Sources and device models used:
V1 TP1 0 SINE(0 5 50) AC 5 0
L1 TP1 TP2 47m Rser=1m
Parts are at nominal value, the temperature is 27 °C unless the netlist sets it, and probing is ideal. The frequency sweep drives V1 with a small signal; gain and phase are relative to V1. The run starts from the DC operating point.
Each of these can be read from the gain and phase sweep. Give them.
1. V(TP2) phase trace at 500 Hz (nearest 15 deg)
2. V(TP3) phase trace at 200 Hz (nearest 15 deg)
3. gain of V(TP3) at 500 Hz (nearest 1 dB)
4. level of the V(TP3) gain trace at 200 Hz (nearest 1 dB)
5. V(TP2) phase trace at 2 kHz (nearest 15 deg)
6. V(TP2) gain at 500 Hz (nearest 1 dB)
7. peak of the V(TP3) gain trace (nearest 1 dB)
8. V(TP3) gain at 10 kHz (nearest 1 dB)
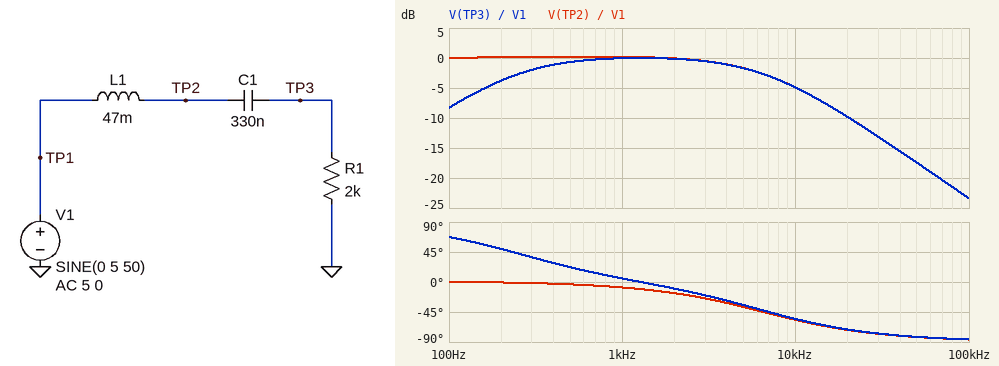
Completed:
0 deg
45 deg
-1 dB
-4 dB
-15 deg
0 dB
0 dB
-5 dB
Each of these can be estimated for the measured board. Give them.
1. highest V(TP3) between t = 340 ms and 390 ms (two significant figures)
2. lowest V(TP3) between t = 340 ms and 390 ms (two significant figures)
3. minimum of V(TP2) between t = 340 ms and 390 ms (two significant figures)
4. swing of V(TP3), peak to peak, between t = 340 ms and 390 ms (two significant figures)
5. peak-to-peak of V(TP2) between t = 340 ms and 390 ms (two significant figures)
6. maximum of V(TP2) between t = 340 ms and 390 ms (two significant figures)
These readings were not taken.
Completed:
1.0 V
-1.0 V
-5.0 V
2.0 V
10 V
5.0 V
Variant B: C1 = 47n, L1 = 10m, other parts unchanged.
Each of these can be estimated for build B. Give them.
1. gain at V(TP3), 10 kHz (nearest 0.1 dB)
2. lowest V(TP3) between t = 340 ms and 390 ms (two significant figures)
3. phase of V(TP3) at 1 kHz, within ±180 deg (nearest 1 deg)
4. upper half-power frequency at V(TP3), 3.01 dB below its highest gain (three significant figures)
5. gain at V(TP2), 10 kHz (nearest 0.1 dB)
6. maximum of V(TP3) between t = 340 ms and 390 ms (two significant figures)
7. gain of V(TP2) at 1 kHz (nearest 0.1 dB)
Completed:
-0.1 dB
-150 mV
59 deg
33.4 kHz
0 dB
150 mV
0.1 dB
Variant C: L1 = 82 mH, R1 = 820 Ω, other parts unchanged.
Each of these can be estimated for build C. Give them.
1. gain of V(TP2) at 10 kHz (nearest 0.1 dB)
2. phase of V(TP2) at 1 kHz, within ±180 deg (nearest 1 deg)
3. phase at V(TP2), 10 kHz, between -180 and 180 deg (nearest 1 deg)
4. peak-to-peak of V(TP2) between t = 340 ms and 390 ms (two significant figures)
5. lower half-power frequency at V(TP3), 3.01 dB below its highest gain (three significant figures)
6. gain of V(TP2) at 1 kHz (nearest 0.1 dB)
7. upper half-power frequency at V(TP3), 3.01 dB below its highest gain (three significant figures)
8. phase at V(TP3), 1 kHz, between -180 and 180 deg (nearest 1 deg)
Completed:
-16.0 dB
-33 deg
-84 deg
10 V
457 Hz
1.3 dB
2.05 kHz
-2 deg
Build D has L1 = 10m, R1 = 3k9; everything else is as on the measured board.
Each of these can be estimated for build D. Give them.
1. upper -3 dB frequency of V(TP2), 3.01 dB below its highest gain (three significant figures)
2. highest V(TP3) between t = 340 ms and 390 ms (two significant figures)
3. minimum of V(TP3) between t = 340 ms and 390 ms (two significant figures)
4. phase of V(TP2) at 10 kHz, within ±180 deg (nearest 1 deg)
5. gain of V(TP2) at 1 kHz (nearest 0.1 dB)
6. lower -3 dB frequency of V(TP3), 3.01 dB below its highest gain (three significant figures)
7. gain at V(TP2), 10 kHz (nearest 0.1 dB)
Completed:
62.0 kHz
1.9 V
-1.9 V
-9 deg
0 dB
123 Hz
-0.1 dB
